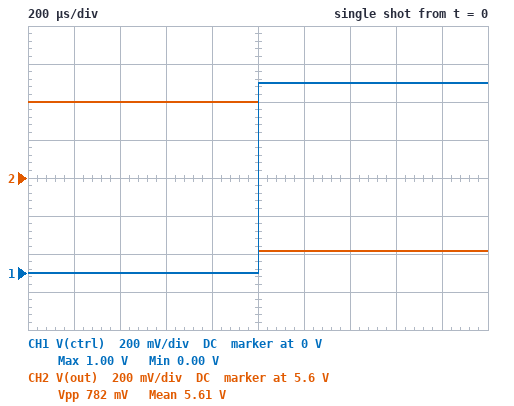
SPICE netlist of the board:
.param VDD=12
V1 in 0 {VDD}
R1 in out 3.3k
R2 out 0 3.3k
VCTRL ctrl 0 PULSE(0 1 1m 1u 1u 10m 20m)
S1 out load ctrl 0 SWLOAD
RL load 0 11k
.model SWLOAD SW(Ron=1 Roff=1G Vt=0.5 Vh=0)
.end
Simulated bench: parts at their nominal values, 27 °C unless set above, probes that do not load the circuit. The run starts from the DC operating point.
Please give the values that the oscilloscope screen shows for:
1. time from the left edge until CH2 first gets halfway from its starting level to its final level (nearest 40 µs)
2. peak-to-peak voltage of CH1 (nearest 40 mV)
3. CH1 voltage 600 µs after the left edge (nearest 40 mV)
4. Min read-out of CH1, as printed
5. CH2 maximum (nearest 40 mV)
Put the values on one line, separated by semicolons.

1.00 ms; 1.00 V; 0 V; 0.00 V; 6.00 V
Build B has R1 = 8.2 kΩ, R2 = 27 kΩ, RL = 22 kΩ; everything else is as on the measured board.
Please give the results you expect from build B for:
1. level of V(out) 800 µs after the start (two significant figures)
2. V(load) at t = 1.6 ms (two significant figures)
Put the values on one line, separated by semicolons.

9.2 V; 7.2 V
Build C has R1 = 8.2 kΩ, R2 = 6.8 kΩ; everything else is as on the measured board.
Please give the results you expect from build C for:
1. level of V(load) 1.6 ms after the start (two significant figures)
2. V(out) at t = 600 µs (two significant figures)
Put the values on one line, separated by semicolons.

4.1 V; 5.4 V
